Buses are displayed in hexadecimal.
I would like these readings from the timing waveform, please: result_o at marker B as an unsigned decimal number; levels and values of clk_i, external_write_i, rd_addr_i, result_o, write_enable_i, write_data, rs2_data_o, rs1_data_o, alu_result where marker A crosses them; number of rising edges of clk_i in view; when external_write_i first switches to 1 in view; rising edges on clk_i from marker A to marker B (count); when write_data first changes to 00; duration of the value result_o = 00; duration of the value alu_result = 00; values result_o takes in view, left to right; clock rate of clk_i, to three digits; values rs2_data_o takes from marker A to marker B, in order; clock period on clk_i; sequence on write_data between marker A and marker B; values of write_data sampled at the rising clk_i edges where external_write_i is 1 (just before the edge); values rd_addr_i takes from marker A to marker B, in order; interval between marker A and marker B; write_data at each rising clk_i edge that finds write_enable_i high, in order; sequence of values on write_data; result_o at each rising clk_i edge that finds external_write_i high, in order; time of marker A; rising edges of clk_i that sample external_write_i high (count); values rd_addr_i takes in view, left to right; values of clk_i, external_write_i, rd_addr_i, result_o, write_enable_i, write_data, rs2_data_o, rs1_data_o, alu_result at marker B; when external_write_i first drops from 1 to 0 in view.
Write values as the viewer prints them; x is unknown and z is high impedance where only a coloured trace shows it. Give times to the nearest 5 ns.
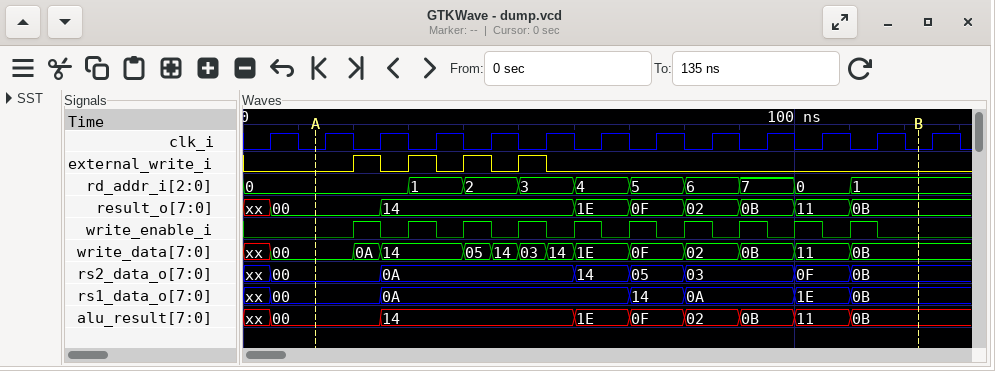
11
clk_i=0, external_write_i=0, rd_addr_i=0, result_o=00, write_enable_i=0, write_data=00, rs2_data_o=00, rs1_data_o=00, alu_result=00
13
20 ns
11
5 ns
20 ns
20 ns
xx, 00, 14, 1E, 0F, 02, 0B, 11, 0B
100 MHz
00, 0A, 14, 05, 03, 0F, 0B
10 ns
00, 0A, 14, 05, 14, 03, 14, 1E, 0F, 02, 0B, 11, 0B
0A, 14, 05, 03
0, 1, 2, 3, 4, 5, 6, 7, 0, 1
110 ns
0A, 14, 05, 03, 1E, 0F, 02, 0B, 11, 0B
xx, 00, 0A, 14, 05, 14, 03, 14, 1E, 0F, 02, 0B, 11, 0B
00, 14, 14, 14
15 ns
4
0, 1, 2, 3, 4, 5, 6, 7, 0, 1
clk_i=0, external_write_i=0, rd_addr_i=1, result_o=0B, write_enable_i=0, write_data=0B, rs2_data_o=0B, rs1_data_o=0B, alu_result=0B
25 ns
